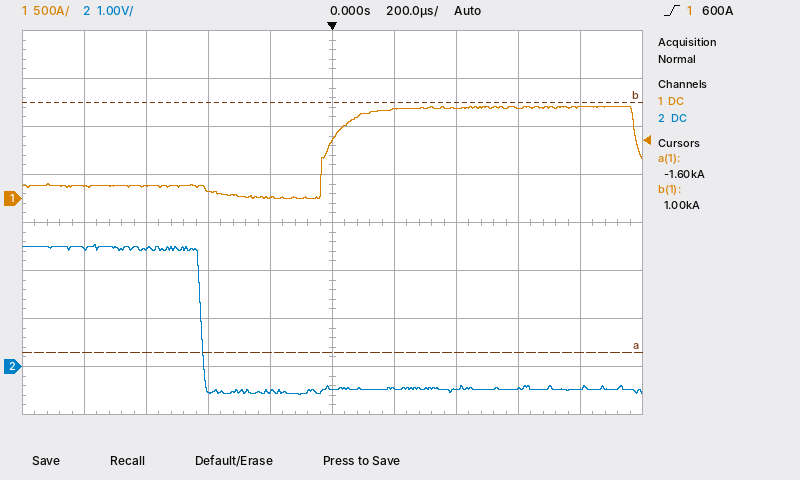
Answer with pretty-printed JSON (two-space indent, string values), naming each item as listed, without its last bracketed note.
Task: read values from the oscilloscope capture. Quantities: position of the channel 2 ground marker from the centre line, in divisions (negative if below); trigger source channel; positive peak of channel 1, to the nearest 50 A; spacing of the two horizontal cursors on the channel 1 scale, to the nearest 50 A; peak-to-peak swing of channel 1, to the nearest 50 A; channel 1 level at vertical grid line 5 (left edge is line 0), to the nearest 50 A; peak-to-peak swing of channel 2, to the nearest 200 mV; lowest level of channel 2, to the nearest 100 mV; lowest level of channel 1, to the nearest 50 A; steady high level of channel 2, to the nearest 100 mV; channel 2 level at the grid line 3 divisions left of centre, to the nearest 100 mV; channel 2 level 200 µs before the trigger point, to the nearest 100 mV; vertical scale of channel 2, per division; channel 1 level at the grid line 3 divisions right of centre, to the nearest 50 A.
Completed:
{
  "position of the channel 2 ground marker from the centre line, in divisions": "-3.0 div",
  "trigger source channel": "channel 1",
  "positive peak of channel 1, to the nearest 50 A": "950 A",
  "spacing of the two horizontal cursors on the channel 1 scale, to the nearest 50 A": "2.60 kA",
  "peak-to-peak swing of channel 1, to the nearest 50 A": "950 A",
  "channel 1 level at vertical grid line 5 (left edge is line 0), to the nearest 50 A": "600 A",
  "peak-to-peak swing of channel 2, to the nearest 200 mV": "3.2 V",
  "lowest level of channel 2, to the nearest 100 mV": "-600 mV",
  "lowest level of channel 1, to the nearest 50 A": "0 A",
  "steady high level of channel 2, to the nearest 100 mV": "2.5 V",
  "channel 2 level at the grid line 3 divisions left of centre, to the nearest 100 mV": "2.5 V",
  "channel 2 level 200 µs before the trigger point, to the nearest 100 mV": "-500 mV",
  "vertical scale of channel 2, per division": "1 V",
  "channel 1 level at the grid line 3 divisions right of centre, to the nearest 50 A": "950 A"
}
